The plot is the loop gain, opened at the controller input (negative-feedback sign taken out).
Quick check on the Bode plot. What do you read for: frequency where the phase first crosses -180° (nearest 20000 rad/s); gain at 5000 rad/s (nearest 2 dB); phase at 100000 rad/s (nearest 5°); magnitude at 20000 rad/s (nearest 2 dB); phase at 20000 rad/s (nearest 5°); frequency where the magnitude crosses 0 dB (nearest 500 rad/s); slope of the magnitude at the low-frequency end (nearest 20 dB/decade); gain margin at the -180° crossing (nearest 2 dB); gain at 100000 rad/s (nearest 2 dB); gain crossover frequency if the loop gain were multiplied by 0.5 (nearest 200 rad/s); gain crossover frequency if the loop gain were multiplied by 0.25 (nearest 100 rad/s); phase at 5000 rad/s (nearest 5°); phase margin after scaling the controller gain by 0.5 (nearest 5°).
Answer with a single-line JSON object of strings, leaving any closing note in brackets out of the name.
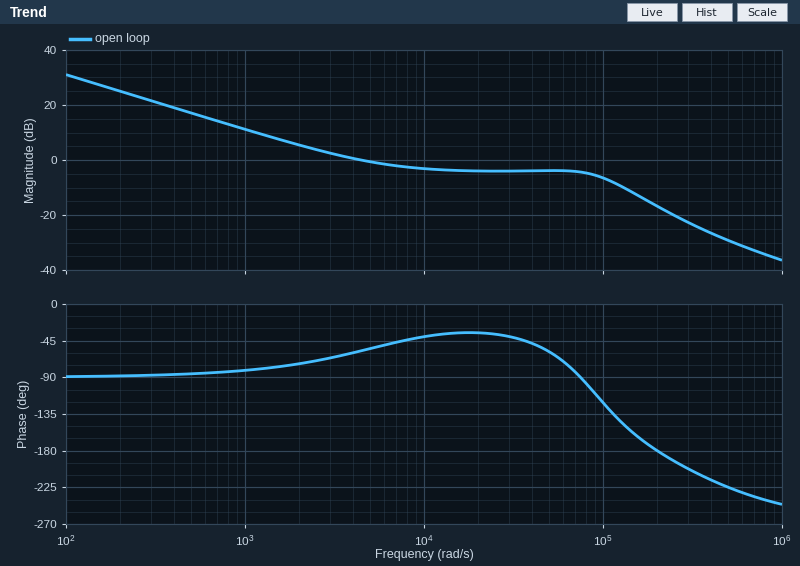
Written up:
{"frequency where the phase first crosses -180°": "200000 rad/s", "gain at 5000 rad/s": "0 dB", "phase at 100000 rad/s": "-120°", "magnitude at 20000 rad/s": "-4 dB", "phase at 20000 rad/s": "-35°", "frequency where the magnitude crosses 0 dB": "4500 rad/s", "slope of the magnitude at the low-frequency end": "-20 dB/decade", "gain margin at the -180° crossing": "16 dB", "gain at 100000 rad/s": "-6 dB", "gain crossover frequency if the loop gain were multiplied by 0.5": "1800 rad/s", "gain crossover frequency if the loop gain were multiplied by 0.25": "900 rad/s", "phase at 5000 rad/s": "-55°", "phase margin after scaling the controller gain by 0.5": "105°"}
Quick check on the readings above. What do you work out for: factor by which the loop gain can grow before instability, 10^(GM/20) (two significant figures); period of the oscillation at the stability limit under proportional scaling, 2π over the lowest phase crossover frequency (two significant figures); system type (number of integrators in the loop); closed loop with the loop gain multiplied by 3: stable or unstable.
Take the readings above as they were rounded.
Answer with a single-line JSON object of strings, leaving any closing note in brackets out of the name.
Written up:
{"factor by which the loop gain can grow before instability, 10^(GM/20)": "6.3", "period of the oscillation at the stability limit under proportional scaling, 2π over the lowest phase crossover frequency": "0.000031 s", "system type": "1", "closed loop with the loop gain multiplied by 3: stable or unstable": "stable"}
